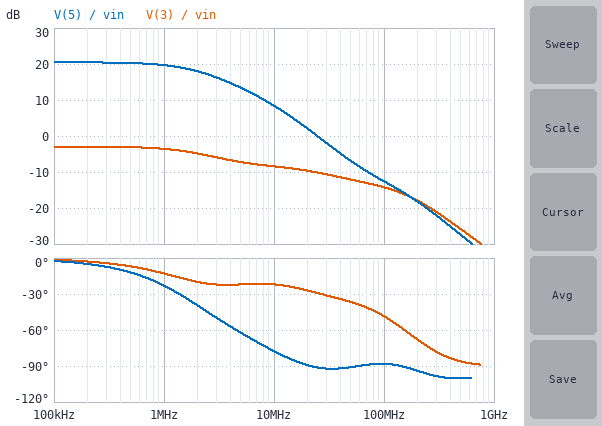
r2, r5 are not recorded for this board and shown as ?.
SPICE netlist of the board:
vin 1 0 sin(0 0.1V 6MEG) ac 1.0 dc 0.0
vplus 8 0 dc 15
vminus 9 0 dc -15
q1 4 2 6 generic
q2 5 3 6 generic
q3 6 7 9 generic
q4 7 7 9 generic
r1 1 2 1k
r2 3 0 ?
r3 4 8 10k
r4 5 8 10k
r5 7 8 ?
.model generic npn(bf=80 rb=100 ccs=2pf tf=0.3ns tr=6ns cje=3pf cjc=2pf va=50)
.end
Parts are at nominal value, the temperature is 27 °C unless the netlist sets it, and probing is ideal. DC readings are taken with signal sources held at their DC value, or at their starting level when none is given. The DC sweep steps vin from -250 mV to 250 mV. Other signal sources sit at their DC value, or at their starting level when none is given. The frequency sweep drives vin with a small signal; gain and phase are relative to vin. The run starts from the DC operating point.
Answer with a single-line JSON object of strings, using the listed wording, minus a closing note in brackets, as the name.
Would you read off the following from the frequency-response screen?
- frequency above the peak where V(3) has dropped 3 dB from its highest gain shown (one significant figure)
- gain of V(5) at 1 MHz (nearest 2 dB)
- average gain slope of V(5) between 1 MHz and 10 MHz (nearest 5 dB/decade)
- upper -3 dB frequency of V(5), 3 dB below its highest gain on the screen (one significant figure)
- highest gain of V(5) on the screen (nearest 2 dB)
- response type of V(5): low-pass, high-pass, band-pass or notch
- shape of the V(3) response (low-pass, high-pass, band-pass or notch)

{"frequency above the peak where V(3) has dropped 3 dB from its highest gain shown": "3 MHz", "gain of V(5) at 1 MHz": "20 dB", "average gain slope of V(5) between 1 MHz and 10 MHz": "-10 dB/decade", "upper -3 dB frequency of V(5), 3 dB below its highest gain on the screen": "2 MHz", "highest gain of V(5) on the screen": "20 dB", "response type of V(5): low-pass, high-pass, band-pass or notch": "low-pass", "shape of the V(3) response": "low-pass"}
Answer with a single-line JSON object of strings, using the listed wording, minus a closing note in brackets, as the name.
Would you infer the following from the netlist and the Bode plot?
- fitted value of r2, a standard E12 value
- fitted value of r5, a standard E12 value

{"fitted value of r2, a standard E12 value": "560 Ω", "fitted value of r5, a standard E12 value": "12 kΩ"}
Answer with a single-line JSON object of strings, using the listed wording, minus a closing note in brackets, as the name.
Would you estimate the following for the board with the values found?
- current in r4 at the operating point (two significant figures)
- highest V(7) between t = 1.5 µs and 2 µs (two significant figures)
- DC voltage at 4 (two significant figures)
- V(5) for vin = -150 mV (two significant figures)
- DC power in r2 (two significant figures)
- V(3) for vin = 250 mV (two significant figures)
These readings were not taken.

{"current in r4 at the operating point": "1.6 mA", "highest V(7) between t = 1.5 µs and 2 µs": "-14 V", "DC voltage at 4": "940 mV", "V(5) for vin = -150 mV": "-880 mV", "DC power in r2": "300 nW", "V(3) for vin = 250 mV": "-7.9 mV"}
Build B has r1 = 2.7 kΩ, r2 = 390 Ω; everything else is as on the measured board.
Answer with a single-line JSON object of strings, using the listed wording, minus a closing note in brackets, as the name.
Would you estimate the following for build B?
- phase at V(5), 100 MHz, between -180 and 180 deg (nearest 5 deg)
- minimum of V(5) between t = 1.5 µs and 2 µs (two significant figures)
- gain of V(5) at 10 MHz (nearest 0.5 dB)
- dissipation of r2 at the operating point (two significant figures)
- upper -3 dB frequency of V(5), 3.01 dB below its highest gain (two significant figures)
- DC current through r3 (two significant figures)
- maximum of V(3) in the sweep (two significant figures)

{"phase at V(5), 100 MHz, between -180 and 180 deg": "-70 deg", "minimum of V(5) between t = 1.5 µs and 2 µs": "-790 mV", "gain of V(5) at 10 MHz": "-6.5 dB", "dissipation of r2 at the operating point": "2.4 µW", "upper -3 dB frequency of V(5), 3.01 dB below its highest gain": "1.7 MHz", "DC current through r3": "1.3 mA", "maximum of V(3) in the sweep": "-6.3 mV"}
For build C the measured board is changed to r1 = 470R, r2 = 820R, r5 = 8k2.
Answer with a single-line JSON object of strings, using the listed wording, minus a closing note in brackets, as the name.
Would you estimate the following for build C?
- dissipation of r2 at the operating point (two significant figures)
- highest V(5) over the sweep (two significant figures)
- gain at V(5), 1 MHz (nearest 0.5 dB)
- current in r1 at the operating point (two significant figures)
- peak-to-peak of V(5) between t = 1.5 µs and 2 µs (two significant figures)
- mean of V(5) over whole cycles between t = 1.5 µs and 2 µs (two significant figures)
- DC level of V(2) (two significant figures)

{"dissipation of r2 at the operating point": "160 µW", "highest V(5) over the sweep": "-1.0 V", "gain at V(5), 1 MHz": "-4.5 dB", "current in r1 at the operating point": "700 µA", "peak-to-peak of V(5) between t = 1.5 µs and 2 µs": "110 mV", "mean of V(5) over whole cycles between t = 1.5 µs and 2 µs": "-1.2 V", "DC level of V(2)": "-330 mV"}
